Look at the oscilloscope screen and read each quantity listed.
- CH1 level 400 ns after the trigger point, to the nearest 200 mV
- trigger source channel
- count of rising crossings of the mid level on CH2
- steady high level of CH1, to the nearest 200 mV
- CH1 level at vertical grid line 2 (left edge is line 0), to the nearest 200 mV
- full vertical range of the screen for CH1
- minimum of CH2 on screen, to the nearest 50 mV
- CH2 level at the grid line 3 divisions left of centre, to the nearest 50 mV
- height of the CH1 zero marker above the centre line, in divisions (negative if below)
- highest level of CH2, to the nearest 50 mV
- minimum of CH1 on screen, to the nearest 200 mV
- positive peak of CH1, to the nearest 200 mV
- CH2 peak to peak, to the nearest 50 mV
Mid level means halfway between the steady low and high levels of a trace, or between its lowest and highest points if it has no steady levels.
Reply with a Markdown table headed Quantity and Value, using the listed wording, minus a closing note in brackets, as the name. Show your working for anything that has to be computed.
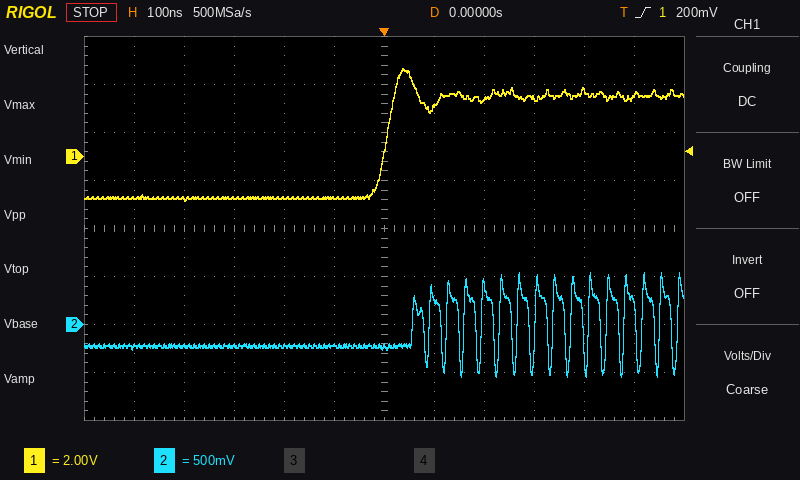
| Quantity | Value |
|---|---|
| CH1 level 400 ns after the trigger point, to the nearest 200 mV | 2.8 V |
| trigger source channel | CH1 |
| count of rising crossings of the mid level on CH2 | 16 |
| steady high level of CH1, to the nearest 200 mV | 2.6 V |
| CH1 level at vertical grid line 2 (left edge is line 0), to the nearest 200 mV | -1.8 V |
| full vertical range of the screen for CH1 | 16 V |
| minimum of CH2 on screen, to the nearest 50 mV | -550 mV |
| CH2 level at the grid line 3 divisions left of centre, to the nearest 50 mV | -200 mV |
| height of the CH1 zero marker above the centre line, in divisions | +1.5 div |
| highest level of CH2, to the nearest 50 mV | 550 mV |
| minimum of CH1 on screen, to the nearest 200 mV | -1.8 V |
| positive peak of CH1, to the nearest 200 mV | 3.6 V |
| CH2 peak to peak, to the nearest 50 mV | 550 mV − (-550 mV) = 1.10 V |
